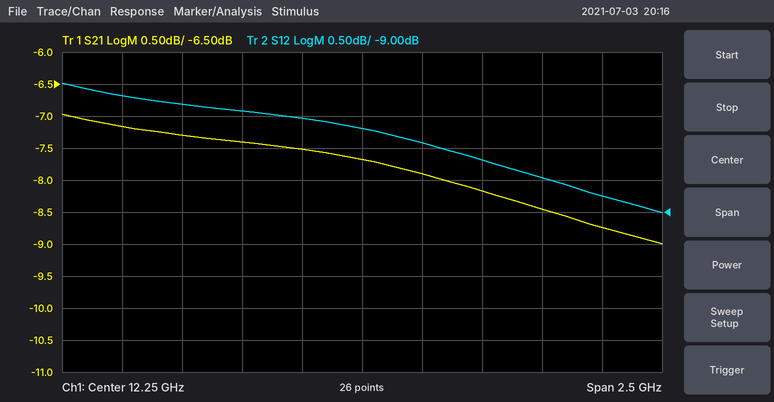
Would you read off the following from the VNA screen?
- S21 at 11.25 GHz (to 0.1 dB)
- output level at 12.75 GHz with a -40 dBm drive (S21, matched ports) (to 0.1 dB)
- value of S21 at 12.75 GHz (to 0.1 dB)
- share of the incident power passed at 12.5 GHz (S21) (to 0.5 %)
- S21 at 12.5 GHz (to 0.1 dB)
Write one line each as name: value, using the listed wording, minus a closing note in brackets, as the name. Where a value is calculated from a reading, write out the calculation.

S21 at 11.25 GHz: -7.2 dB
output level at 12.75 GHz with a -40 dBm drive (S21, matched ports): -40 dBm + (-8.2 dB) = -48.2 dBm
value of S21 at 12.75 GHz: -8.2 dB
share of the incident power passed at 12.5 GHz (S21): 10^(-7.9/10) ≈ 16.2 %, so 16.0 % to the nearest 0.5 %
S21 at 12.5 GHz: -7.9 dB
